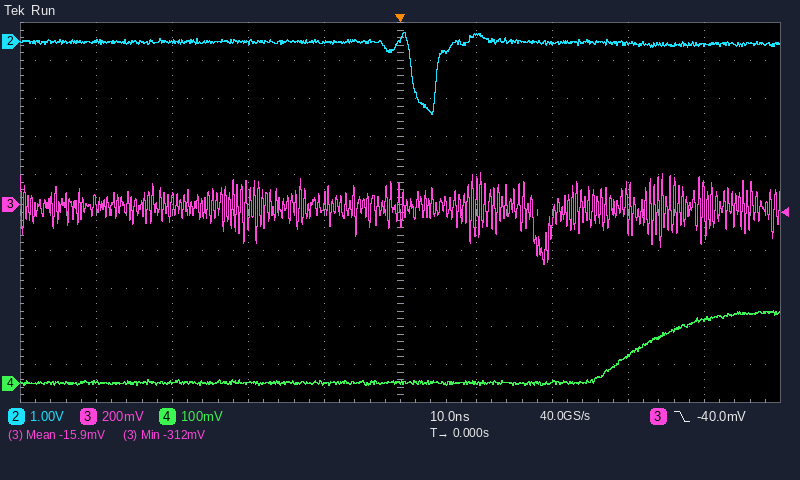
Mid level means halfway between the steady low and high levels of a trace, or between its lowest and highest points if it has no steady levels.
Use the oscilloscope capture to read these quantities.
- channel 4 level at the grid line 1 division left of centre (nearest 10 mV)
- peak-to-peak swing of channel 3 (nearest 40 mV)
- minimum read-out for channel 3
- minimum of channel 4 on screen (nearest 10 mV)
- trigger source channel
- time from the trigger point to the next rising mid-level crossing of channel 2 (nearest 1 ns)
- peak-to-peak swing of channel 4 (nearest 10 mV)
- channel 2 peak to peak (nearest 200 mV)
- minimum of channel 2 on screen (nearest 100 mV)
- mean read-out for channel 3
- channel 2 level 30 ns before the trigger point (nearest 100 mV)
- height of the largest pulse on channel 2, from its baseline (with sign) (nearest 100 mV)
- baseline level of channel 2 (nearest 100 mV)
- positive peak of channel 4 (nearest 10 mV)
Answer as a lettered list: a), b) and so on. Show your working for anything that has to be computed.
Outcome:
a) 0 mV
b) 480 mV
c) -312 mV
d) -10 mV
e) channel 3
f) 5 ns
g) 190 mV − (-10 mV) = 200 mV
h) 2.2 V
i) -1.9 V
j) -15.9 mV
k) 0.0 V
l) -1.9 V − (0.0 V) = -1.9 V
m) 0.0 V
n) 190 mV
